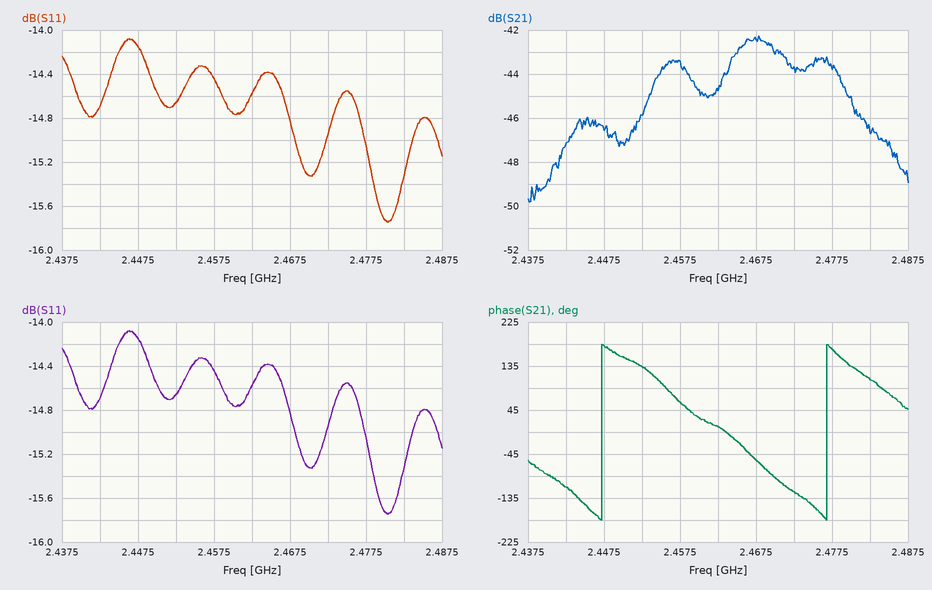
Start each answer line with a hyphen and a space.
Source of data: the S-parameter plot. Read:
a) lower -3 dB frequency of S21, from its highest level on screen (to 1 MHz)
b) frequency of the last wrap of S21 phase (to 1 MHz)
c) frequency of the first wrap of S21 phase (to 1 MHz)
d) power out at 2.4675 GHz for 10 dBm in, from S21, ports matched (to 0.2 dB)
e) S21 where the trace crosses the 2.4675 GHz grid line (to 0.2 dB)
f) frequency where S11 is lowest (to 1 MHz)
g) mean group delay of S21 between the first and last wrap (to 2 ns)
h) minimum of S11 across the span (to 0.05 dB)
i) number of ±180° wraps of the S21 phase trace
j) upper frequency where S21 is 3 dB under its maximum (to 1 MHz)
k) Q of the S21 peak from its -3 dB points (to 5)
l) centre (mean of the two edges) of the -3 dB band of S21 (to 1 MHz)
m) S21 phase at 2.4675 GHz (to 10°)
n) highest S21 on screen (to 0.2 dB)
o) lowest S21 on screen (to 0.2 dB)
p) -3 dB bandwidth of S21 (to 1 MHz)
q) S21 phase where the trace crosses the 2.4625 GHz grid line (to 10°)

- 2.453 GHz
- 2.477 GHz
- 2.447 GHz
- -32.4 dBm
- -42.4 dB
- 2.480 GHz
- 34 ns
- -15.75 dB
- 2
- 2.480 GHz
- 90
- 2.467 GHz
- -60°
- -42.2 dB
- -49.8 dB
- 27 MHz
- 10°
